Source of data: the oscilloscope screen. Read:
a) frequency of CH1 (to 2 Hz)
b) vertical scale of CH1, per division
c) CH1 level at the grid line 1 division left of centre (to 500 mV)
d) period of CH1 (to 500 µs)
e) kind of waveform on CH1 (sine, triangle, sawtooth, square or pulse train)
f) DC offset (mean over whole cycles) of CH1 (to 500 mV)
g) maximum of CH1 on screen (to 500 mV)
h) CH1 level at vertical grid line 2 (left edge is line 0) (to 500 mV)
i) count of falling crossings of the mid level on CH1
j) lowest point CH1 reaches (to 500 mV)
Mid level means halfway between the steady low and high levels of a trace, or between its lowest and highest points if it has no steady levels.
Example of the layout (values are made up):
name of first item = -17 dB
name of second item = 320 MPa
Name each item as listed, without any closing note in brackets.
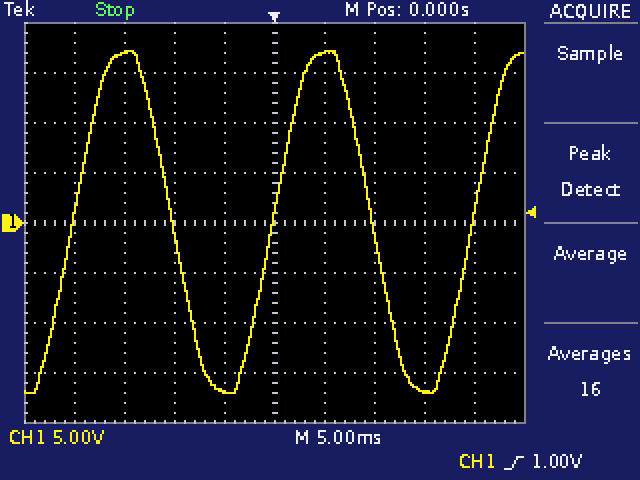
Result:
frequency of CH1 = 50 Hz
vertical scale of CH1, per division = 5 V
CH1 level at the grid line 1 division left of centre = -17.0 V
period of CH1 = 20.0 ms
kind of waveform on CH1 = sine
DC offset (mean over whole cycles) of CH1 = 0.0 V
maximum of CH1 on screen = 17.0 V
CH1 level at vertical grid line 2 (left edge is line 0) = 17.0 V
count of falling crossings of the mid level on CH1 = 2
lowest point CH1 reaches = -17.0 V
